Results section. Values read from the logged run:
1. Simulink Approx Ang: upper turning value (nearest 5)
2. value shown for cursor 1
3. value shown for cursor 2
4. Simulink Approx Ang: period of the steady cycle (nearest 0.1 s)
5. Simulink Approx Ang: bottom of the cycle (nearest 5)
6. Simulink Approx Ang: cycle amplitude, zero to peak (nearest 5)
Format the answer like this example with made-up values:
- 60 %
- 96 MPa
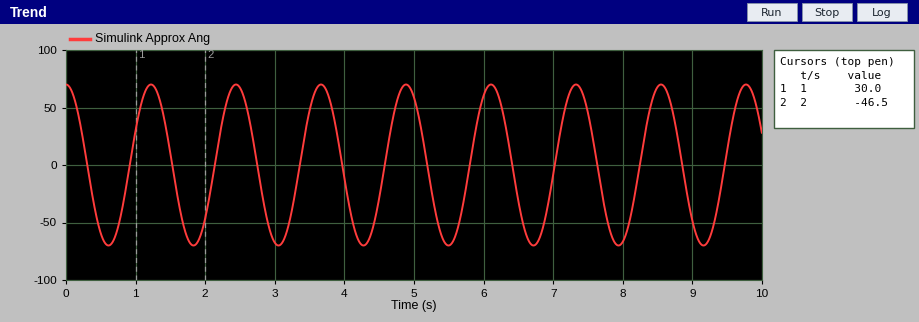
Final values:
- 70
- 30.0
- -46.5
- 1.2 s
- -70
- 70
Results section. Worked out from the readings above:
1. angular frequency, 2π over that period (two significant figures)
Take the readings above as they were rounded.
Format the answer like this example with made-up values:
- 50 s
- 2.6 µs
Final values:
- 5.2 rad/s
